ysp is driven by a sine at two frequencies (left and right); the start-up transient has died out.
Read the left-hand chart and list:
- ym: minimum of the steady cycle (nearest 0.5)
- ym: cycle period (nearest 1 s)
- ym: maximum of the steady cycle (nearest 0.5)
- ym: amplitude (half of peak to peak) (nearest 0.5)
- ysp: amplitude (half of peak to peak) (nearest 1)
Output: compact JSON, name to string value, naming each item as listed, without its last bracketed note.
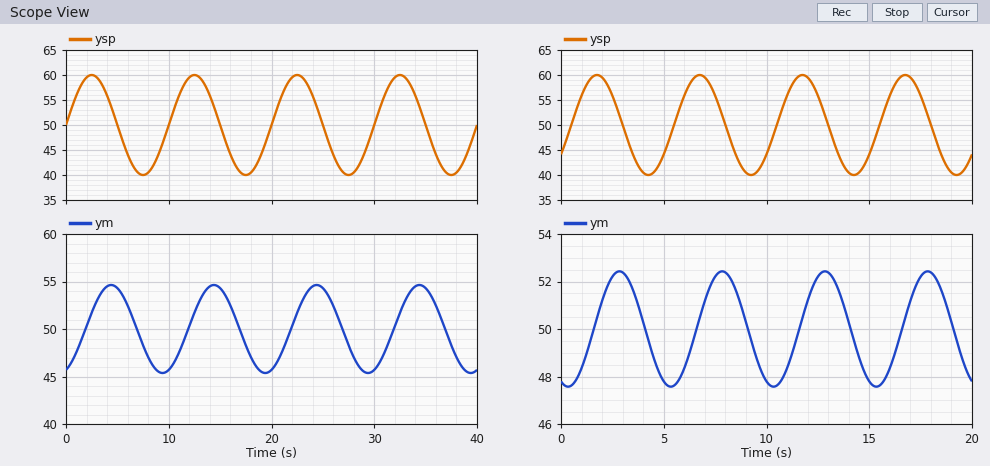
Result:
{"ym: minimum of the steady cycle": "45.5", "ym: cycle period": "10 s", "ym: maximum of the steady cycle": "54.5", "ym: amplitude (half of peak to peak)": "4.5", "ysp: amplitude (half of peak to peak)": "10"}
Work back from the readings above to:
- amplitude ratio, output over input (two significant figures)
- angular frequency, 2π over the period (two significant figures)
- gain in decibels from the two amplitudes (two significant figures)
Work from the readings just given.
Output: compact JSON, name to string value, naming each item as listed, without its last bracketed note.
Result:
{"amplitude ratio, output over input": "0.45", "angular frequency, 2π over the period": "0.63 rad/s", "gain in decibels from the two amplitudes": "-6.9 dB"}
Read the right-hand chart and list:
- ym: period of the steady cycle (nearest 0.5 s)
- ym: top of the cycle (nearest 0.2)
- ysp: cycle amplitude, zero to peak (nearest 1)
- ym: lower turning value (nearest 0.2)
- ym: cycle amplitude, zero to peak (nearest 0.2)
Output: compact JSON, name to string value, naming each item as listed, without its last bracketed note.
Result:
{"ym: period of the steady cycle": "5.0 s", "ym: top of the cycle": "52.4", "ysp: cycle amplitude, zero to peak": "10", "ym: lower turning value": "47.6", "ym: cycle amplitude, zero to peak": "2.4"}
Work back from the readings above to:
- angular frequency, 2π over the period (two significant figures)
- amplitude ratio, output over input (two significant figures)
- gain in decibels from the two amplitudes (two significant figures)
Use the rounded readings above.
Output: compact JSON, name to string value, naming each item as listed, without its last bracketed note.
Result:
{"angular frequency, 2π over the period": "1.3 rad/s", "amplitude ratio, output over input": "0.24", "gain in decibels from the two amplitudes": "-12 dB"}
